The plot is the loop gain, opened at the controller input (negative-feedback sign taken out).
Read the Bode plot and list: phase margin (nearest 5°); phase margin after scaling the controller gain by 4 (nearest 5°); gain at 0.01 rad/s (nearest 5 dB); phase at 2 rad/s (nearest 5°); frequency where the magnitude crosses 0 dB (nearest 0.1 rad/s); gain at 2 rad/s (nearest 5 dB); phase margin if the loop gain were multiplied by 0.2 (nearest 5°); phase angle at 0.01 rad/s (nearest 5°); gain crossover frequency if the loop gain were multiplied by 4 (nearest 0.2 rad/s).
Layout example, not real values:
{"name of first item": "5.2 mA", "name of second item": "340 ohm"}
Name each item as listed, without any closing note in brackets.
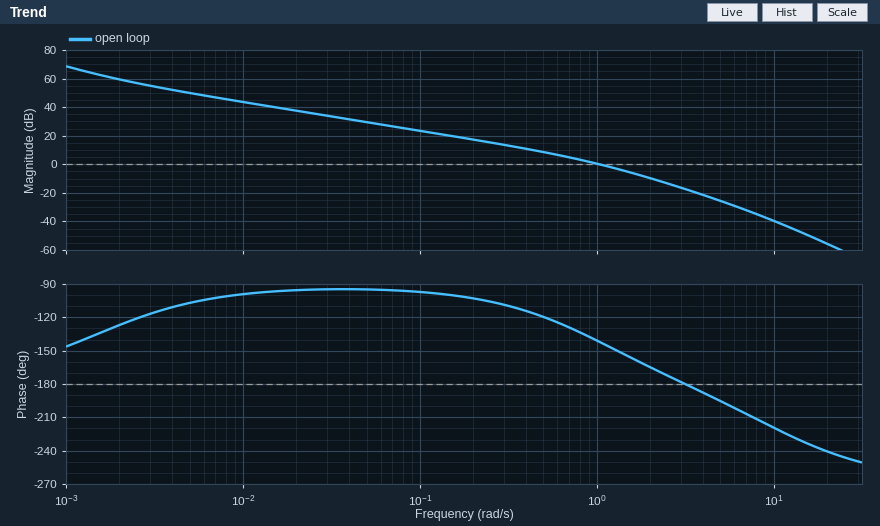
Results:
{"phase margin": "40°", "phase margin after scaling the controller gain by 4": "10°", "gain at 0.01 rad/s": "45 dB", "phase at 2 rad/s": "-165°", "frequency where the magnitude crosses 0 dB": "1.0 rad/s", "gain at 2 rad/s": "-10 dB", "phase margin if the loop gain were multiplied by 0.2": "70°", "phase angle at 0.01 rad/s": "-100°", "gain crossover frequency if the loop gain were multiplied by 4": "2.4 rad/s"}
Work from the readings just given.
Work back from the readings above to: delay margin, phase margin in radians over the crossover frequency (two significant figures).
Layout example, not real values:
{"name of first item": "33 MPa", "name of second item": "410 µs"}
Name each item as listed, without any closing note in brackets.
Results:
{"delay margin, phase margin in radians over the crossover frequency": "0.70 s"}
